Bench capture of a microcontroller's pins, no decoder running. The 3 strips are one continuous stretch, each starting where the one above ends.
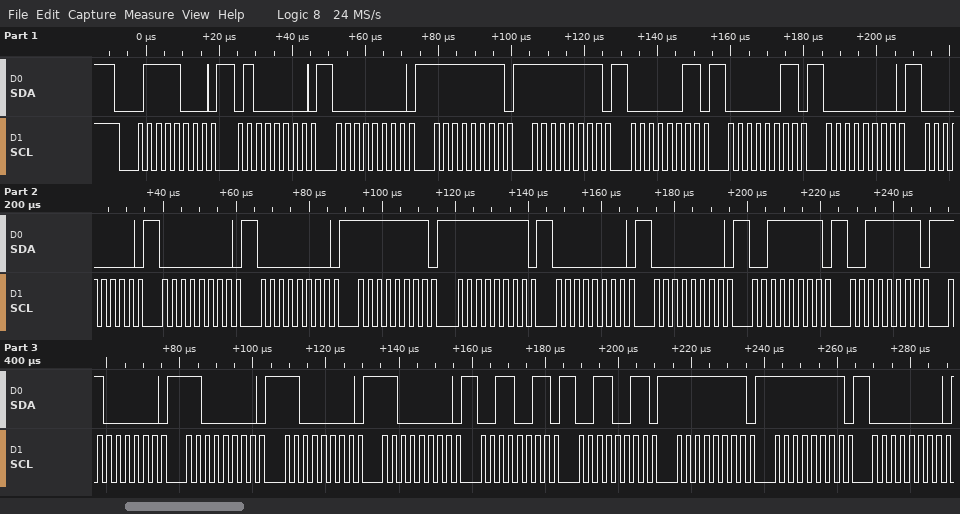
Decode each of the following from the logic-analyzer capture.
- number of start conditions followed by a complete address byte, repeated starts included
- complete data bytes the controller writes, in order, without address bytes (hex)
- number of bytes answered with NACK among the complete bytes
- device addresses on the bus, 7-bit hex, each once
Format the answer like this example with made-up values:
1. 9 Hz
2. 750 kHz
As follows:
1. 1
2. 40 00 FF FF 03 03 00 00 00 00 FF FF 00 00 3F 3F C0 C0 C0 C0 33 33 FF FF 00
3. 0
4. 0x3C
